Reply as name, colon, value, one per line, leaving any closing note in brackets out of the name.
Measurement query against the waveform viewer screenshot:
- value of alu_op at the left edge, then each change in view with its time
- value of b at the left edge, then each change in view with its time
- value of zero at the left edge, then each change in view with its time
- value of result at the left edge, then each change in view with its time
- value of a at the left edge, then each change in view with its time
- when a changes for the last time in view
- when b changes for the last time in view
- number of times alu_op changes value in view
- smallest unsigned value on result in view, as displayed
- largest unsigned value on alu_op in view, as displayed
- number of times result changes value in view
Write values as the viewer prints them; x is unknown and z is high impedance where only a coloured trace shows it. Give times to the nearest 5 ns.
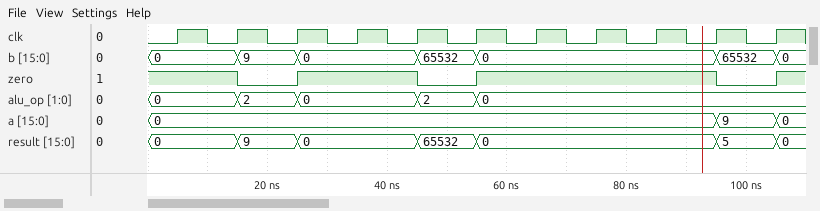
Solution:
value of alu_op at the left edge, then each change in view with its time: 0, 2 at 15 ns, 0 at 25 ns, 2 at 45 ns, 0 at 55 ns
value of b at the left edge, then each change in view with its time: 0, 9 at 15 ns, 0 at 25 ns, 65532 at 45 ns, 0 at 55 ns, 65532 at 95 ns, 0 at 105 ns
value of zero at the left edge, then each change in view with its time: 1, 0 at 15 ns, 1 at 25 ns, 0 at 45 ns, 1 at 55 ns, 0 at 95 ns, 1 at 105 ns
value of result at the left edge, then each change in view with its time: 0, 9 at 15 ns, 0 at 25 ns, 65532 at 45 ns, 0 at 55 ns, 5 at 95 ns, 0 at 105 ns
value of a at the left edge, then each change in view with its time: 0, 9 at 95 ns, 0 at 105 ns
when a changes for the last time in view: 105 ns
when b changes for the last time in view: 105 ns
number of times alu_op changes value in view: 4
smallest unsigned value on result in view, as displayed: 0
largest unsigned value on alu_op in view, as displayed: 2
number of times result changes value in view: 6
